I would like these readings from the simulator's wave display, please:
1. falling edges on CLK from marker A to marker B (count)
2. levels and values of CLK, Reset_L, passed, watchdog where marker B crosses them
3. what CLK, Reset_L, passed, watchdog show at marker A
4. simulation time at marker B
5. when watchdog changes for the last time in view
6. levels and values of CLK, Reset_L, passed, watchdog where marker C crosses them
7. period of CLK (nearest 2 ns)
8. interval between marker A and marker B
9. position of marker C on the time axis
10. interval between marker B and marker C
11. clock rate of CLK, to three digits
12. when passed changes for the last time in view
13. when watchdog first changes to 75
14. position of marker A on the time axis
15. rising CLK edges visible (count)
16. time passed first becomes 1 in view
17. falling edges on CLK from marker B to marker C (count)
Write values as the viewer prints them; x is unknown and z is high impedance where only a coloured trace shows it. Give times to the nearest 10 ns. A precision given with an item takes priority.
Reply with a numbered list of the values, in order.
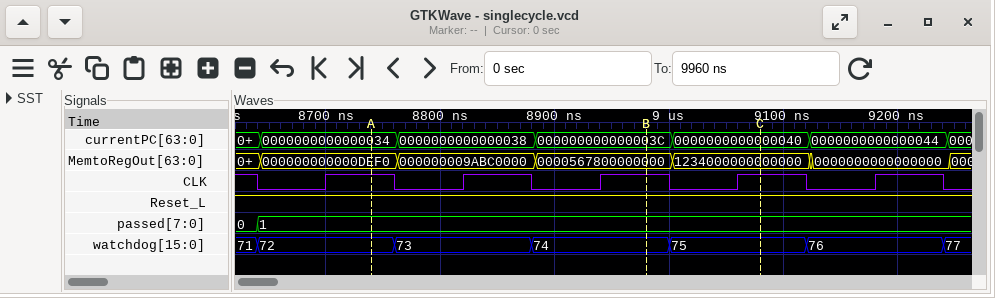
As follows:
1. 2
2. CLK=1, Reset_L=1, passed=1, watchdog=74
3. CLK=1, Reset_L=1, passed=1, watchdog=72
4. 8980 ns
5. 9240 ns
6. CLK=1, Reset_L=1, passed=1, watchdog=75
7. 120 ns
8. 240 ns
9. 9080 ns
10. 100 ns
11. 8.33 MHz
12. 8640 ns
13. 9000 ns
14. 8740 ns
15. 5
16. 8640 ns
17. 1
